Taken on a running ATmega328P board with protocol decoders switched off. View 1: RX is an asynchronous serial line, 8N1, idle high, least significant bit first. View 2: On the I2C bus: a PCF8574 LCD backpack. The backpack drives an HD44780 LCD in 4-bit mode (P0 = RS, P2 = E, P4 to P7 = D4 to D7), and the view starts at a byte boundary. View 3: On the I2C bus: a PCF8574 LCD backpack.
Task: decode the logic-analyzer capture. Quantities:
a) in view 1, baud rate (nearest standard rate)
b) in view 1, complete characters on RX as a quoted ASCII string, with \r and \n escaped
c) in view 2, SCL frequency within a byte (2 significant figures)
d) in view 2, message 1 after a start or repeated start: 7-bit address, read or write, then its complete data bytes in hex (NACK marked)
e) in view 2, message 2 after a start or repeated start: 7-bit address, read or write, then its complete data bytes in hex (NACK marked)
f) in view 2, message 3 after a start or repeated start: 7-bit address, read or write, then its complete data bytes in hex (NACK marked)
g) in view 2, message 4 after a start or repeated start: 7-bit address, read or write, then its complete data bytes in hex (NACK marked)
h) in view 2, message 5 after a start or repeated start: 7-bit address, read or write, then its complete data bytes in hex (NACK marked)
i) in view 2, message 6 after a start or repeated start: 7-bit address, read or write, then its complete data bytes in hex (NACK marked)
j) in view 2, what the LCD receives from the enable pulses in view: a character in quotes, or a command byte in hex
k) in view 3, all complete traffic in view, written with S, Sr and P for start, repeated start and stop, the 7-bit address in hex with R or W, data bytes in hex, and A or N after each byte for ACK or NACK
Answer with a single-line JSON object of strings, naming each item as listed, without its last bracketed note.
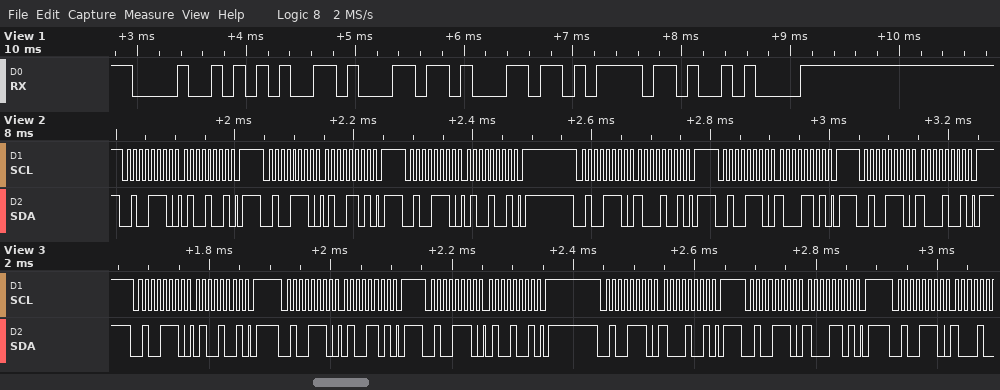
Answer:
{"in view 1, baud rate": "9600 baud", "in view 1, complete characters on RX as a quoted ASCII string, with \\r and \\n escaped": "\"Hello\\n\"", "in view 2, SCL frequency within a byte": "100 kHz", "in view 2, message 1 after a start or repeated start: 7-bit address, read or write, then its complete data bytes in hex": "0x27 write: 49", "in view 2, message 2 after a start or repeated start: 7-bit address, read or write, then its complete data bytes in hex": "0x27 write: 4D", "in view 2, message 3 after a start or repeated start: 7-bit address, read or write, then its complete data bytes in hex": "0x27 write: 49", "in view 2, message 4 after a start or repeated start: 7-bit address, read or write, then its complete data bytes in hex": "0x27 write: 89", "in view 2, message 5 after a start or repeated start: 7-bit address, read or write, then its complete data bytes in hex": "0x27 write: 8D", "in view 2, message 6 after a start or repeated start: 7-bit address, read or write, then its complete data bytes in hex": "0x27 write: 89", "in view 2, what the LCD receives from the enable pulses in view: a character in quotes, or a command byte in hex": "'H'", "in view 3, all complete traffic in view, written with S, Sr and P for start, repeated start and stop, the 7-bit address in hex with R or W, data bytes in hex, and A or N after each byte for ACK or NACK": "S 27W A 49 A P S 27W A 4D A P S 27W A 49 A P S 27W A 89 A P S 27W A 8D A P S 27W A"}
